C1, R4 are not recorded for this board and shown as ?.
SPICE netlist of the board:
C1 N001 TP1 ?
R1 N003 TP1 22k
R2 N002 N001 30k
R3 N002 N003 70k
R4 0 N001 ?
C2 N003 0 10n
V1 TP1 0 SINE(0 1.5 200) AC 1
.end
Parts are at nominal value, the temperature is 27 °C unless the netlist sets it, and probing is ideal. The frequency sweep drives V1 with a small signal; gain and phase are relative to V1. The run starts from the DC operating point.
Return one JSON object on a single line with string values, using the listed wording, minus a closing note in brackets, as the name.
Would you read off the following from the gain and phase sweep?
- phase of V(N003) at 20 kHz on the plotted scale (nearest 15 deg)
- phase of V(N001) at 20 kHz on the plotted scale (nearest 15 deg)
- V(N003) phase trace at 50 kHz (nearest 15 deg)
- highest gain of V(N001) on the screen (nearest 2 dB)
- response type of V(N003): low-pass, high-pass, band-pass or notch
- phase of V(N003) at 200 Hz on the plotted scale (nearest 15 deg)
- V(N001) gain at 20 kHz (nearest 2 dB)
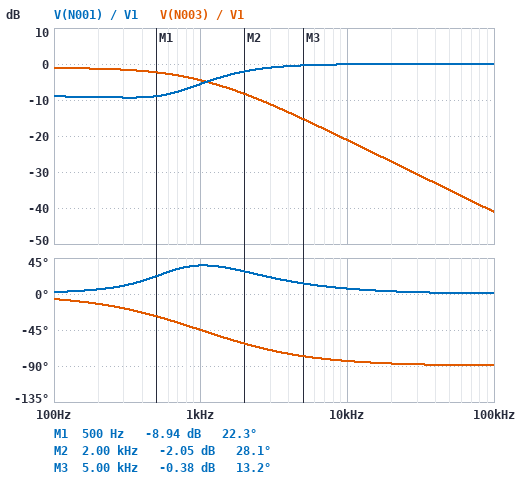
{"phase of V(N003) at 20 kHz on the plotted scale": "-90 deg", "phase of V(N001) at 20 kHz on the plotted scale": "0 deg", "V(N003) phase trace at 50 kHz": "-90 deg", "highest gain of V(N001) on the screen": "0 dB", "response type of V(N003): low-pass, high-pass, band-pass or notch": "low-pass", "phase of V(N003) at 200 Hz on the plotted scale": "-15 deg", "V(N001) gain at 20 kHz": "0 dB"}
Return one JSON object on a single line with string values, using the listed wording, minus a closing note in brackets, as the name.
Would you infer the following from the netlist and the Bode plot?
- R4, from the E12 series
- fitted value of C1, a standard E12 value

{"R4, from the E12 series": "68 kΩ", "fitted value of C1, a standard E12 value": "3.3 nF"}
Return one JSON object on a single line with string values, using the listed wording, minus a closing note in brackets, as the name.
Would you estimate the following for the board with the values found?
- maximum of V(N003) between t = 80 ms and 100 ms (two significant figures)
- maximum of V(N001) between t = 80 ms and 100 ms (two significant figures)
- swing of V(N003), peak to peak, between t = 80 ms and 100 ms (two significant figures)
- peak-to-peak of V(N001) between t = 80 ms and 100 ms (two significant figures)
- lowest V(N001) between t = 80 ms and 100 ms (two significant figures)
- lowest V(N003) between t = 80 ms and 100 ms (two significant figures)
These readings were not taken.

{"maximum of V(N003) between t = 80 ms and 100 ms": "1.3 V", "maximum of V(N001) between t = 80 ms and 100 ms": "520 mV", "swing of V(N003), peak to peak, between t = 80 ms and 100 ms": "2.6 V", "peak-to-peak of V(N001) between t = 80 ms and 100 ms": "1.0 V", "lowest V(N001) between t = 80 ms and 100 ms": "-520 mV", "lowest V(N003) between t = 80 ms and 100 ms": "-1.3 V"}
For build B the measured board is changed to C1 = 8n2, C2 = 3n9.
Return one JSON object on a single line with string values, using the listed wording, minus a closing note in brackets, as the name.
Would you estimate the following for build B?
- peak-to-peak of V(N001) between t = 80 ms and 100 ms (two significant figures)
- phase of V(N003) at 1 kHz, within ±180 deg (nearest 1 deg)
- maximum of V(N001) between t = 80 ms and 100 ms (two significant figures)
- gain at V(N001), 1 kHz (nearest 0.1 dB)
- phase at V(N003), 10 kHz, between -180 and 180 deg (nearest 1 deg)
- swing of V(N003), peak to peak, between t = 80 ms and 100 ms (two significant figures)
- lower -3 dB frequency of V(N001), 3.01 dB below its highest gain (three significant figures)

{"peak-to-peak of V(N001) between t = 80 ms and 100 ms": "1.5 V", "phase of V(N003) at 1 kHz, within ±180 deg": "-21 deg", "maximum of V(N001) between t = 80 ms and 100 ms": "750 mV", "gain at V(N001), 1 kHz": "-1.3 dB", "phase at V(N003), 10 kHz, between -180 and 180 deg": "-77 deg", "swing of V(N003), peak to peak, between t = 80 ms and 100 ms": "2.7 V", "lower -3 dB frequency of V(N001), 3.01 dB below its highest gain": "463 Hz"}
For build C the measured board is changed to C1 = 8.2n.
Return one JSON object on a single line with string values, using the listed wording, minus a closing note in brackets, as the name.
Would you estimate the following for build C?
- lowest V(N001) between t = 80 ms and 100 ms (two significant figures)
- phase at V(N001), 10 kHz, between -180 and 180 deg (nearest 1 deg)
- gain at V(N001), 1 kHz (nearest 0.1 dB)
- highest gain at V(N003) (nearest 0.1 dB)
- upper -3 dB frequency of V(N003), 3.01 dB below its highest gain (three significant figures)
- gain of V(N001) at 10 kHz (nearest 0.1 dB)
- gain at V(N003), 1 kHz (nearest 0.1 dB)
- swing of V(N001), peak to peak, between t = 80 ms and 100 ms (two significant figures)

{"lowest V(N001) between t = 80 ms and 100 ms": "-680 mV", "phase at V(N001), 10 kHz, between -180 and 180 deg": "3 deg", "gain at V(N001), 1 kHz": "-1.7 dB", "highest gain at V(N003)": "-1.1 dB", "upper -3 dB frequency of V(N003), 3.01 dB below its highest gain": "1.03 kHz", "gain of V(N001) at 10 kHz": "0 dB", "gain at V(N003), 1 kHz": "-3.9 dB", "swing of V(N001), peak to peak, between t = 80 ms and 100 ms": "1.4 V"}
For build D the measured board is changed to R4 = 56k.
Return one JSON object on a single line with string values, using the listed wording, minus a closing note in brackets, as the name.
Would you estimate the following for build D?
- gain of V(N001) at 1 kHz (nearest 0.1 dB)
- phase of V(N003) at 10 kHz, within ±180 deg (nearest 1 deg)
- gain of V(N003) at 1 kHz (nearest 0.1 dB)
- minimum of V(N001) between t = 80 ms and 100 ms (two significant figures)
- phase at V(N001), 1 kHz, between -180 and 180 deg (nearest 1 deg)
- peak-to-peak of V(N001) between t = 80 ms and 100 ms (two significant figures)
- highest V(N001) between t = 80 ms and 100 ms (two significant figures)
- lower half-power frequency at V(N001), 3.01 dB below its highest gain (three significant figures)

{"gain of V(N001) at 1 kHz": "-6.2 dB", "phase of V(N003) at 10 kHz, within ±180 deg": "-84 deg", "gain of V(N003) at 1 kHz": "-4.6 dB", "minimum of V(N001) between t = 80 ms and 100 ms": "-460 mV", "phase at V(N001), 1 kHz, between -180 and 180 deg": "39 deg", "peak-to-peak of V(N001) between t = 80 ms and 100 ms": "920 mV", "highest V(N001) between t = 80 ms and 100 ms": "460 mV", "lower half-power frequency at V(N001), 3.01 dB below its highest gain": "1.71 kHz"}
